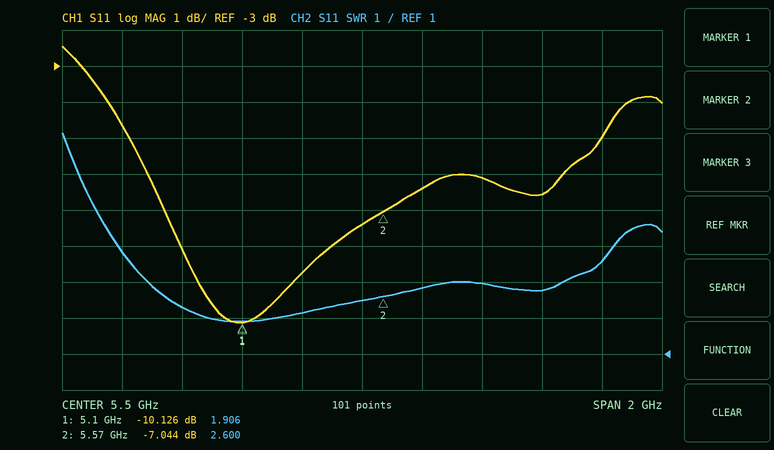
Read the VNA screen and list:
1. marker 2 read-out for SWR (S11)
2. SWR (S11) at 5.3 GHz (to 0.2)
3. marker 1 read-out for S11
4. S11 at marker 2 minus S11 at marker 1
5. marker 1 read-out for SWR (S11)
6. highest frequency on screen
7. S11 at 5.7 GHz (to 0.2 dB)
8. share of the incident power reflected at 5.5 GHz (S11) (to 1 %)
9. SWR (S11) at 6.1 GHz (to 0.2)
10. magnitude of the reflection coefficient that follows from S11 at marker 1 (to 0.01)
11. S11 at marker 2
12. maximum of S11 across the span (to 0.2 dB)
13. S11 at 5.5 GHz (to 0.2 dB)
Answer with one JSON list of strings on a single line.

["2.600", "2.2", "-10.126 dB", "3.082 dB", "1.906", "6.5 GHz", "-6.4 dB", "18 %", "2.8", "0.31", "-7.044 dB", "-2.4 dB", "-7.4 dB"]
